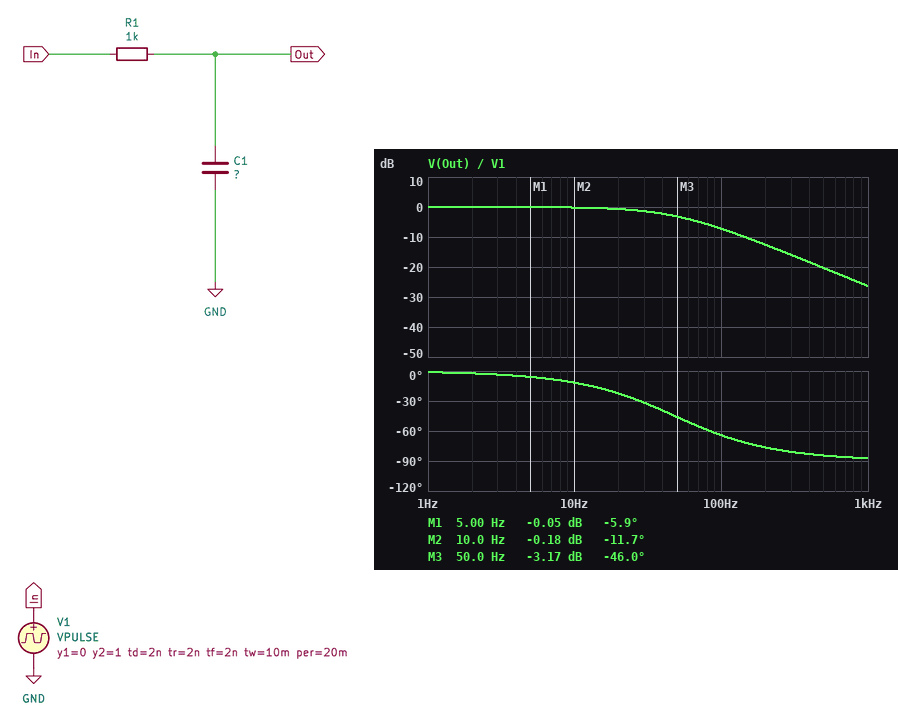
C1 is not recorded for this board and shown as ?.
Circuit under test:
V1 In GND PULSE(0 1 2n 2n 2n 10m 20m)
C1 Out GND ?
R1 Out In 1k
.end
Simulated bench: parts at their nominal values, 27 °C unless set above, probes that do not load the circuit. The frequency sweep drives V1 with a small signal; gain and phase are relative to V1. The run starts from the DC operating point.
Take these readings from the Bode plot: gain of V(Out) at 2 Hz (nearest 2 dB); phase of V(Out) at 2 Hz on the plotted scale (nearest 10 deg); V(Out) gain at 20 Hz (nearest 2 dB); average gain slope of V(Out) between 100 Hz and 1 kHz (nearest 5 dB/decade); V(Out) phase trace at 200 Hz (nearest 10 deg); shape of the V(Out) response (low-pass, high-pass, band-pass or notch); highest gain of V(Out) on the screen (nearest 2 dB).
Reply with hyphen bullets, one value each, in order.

- 0 dB
- 0 deg
- 0 dB
- -20 dB/decade
- -80 deg
- low-pass
- 0 dB
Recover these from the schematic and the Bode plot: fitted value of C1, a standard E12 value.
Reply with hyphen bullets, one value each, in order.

- 3.3 µF
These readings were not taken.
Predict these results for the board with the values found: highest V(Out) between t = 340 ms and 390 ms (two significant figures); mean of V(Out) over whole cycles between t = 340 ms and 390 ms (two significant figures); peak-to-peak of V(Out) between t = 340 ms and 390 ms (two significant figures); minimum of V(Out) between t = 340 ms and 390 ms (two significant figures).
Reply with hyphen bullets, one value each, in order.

- 950 mV
- 500 mV
- 910 mV
- 46 mV
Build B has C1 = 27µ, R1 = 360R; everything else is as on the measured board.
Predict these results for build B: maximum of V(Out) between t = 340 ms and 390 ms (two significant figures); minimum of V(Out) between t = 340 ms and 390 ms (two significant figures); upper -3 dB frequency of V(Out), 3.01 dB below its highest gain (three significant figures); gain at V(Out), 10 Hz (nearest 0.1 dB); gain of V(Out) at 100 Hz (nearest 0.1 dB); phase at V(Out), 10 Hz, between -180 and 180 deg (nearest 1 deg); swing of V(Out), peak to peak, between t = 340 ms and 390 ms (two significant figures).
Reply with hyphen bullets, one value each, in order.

- 740 mV
- 260 mV
- 16.4 Hz
- -1.4 dB
- -15.8 dB
- -31 deg
- 470 mV
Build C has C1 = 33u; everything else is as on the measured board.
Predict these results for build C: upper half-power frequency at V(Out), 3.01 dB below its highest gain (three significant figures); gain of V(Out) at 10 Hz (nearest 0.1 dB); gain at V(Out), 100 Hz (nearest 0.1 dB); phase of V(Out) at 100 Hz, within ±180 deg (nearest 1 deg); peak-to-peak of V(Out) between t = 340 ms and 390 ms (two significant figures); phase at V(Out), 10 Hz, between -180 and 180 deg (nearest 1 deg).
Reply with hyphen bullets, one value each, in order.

- 4.82 Hz
- -7.2 dB
- -26.3 dB
- -87 deg
- 150 mV
- -64 deg
